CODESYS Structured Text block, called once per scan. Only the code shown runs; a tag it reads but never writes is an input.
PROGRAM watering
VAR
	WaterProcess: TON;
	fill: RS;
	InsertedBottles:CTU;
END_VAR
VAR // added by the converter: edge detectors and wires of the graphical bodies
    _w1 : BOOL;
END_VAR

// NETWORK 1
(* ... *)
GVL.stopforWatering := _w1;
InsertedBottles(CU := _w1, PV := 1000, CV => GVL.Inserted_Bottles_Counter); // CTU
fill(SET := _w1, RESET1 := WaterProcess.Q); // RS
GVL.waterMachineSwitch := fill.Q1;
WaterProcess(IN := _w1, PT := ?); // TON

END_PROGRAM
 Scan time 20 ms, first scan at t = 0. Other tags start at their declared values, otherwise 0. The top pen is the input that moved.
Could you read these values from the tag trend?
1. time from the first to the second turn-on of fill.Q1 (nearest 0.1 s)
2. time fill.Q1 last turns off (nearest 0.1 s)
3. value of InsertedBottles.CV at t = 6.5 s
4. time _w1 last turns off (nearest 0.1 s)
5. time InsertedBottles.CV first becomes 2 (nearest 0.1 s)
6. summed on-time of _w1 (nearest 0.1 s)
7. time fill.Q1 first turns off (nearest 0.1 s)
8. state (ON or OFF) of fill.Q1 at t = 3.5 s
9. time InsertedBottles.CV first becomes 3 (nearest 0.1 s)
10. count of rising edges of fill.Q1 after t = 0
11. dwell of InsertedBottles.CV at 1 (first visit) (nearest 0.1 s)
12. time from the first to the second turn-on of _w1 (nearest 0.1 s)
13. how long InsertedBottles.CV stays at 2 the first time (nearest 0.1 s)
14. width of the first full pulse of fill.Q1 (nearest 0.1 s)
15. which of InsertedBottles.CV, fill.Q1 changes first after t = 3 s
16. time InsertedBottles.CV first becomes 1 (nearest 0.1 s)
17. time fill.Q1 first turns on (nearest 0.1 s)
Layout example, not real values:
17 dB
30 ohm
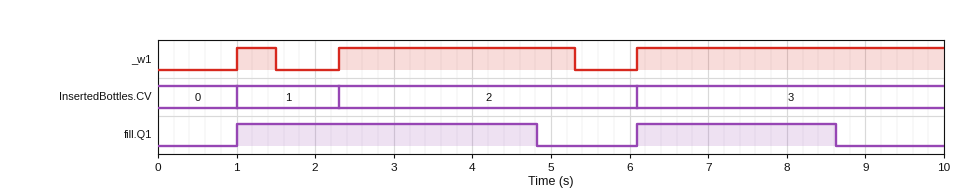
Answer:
5.1 s
8.6 s
3
5.3 s
2.3 s
7.4 s
4.8 s
ON
6.1 s
2
1.3 s
1.3 s
3.8 s
3.8 s
fill.Q1
1.0 s
1.0 s
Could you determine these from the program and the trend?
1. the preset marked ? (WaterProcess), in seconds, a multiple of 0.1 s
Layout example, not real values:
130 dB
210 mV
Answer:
2.5 s
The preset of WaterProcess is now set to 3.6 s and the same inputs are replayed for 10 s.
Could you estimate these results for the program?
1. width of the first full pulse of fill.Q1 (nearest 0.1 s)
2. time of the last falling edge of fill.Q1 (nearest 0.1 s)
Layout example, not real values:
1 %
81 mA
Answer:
8.7 s
9.7 s
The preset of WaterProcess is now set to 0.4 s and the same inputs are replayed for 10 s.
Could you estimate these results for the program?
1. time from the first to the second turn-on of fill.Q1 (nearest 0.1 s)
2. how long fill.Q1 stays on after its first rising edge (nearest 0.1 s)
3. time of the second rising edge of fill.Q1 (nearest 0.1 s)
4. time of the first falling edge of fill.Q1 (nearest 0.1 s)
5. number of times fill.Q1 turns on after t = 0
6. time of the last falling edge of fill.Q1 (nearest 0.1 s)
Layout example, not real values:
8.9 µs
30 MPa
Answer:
1.3 s
0.4 s
2.3 s
1.4 s
3
6.5 s
